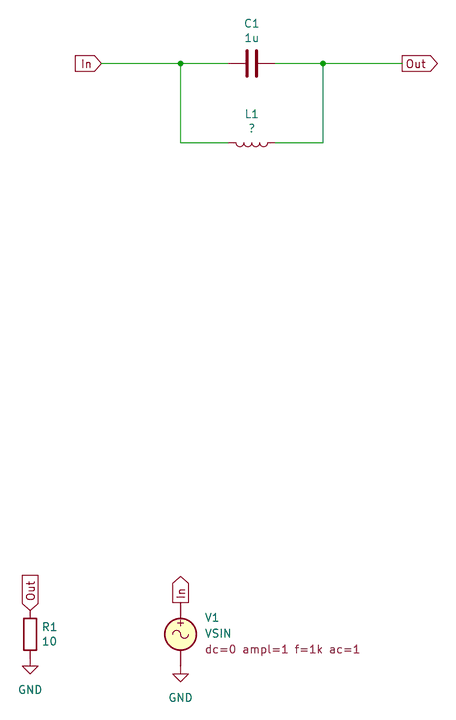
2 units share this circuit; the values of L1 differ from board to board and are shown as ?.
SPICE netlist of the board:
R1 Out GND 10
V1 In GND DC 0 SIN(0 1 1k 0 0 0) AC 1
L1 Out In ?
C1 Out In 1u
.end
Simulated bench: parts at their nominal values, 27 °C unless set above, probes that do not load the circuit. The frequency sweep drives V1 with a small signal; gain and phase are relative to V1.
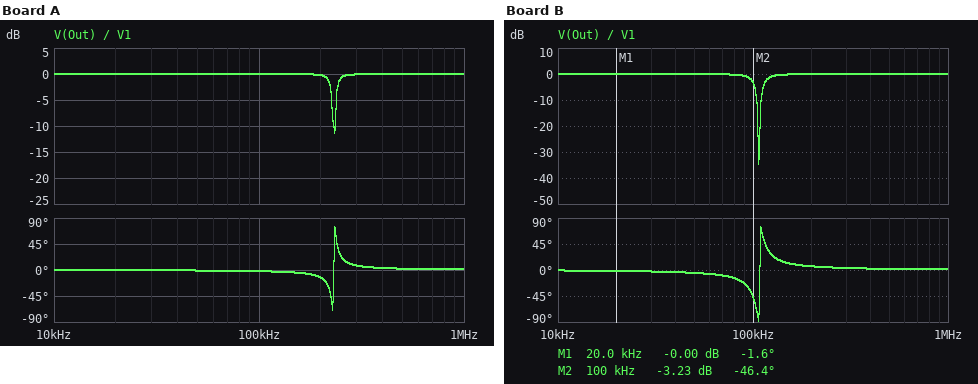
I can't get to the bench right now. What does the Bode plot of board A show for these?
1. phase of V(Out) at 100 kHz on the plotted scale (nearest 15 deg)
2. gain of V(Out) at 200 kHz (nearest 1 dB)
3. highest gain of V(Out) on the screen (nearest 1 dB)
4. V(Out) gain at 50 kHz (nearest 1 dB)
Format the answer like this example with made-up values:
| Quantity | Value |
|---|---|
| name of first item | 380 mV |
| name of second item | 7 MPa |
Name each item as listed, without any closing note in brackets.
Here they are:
| Quantity | Value |
|---|---|
| phase of V(Out) at 100 kHz on the plotted scale | 0 deg |
| gain of V(Out) at 200 kHz | 0 dB |
| highest gain of V(Out) on the screen | 0 dB |
| V(Out) gain at 50 kHz | 0 dB |
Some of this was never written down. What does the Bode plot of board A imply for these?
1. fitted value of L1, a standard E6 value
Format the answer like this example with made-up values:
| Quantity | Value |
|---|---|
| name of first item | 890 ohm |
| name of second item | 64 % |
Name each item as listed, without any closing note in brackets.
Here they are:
| Quantity | Value |
|---|---|
| fitted value of L1, a standard E6 value | 470 nH |
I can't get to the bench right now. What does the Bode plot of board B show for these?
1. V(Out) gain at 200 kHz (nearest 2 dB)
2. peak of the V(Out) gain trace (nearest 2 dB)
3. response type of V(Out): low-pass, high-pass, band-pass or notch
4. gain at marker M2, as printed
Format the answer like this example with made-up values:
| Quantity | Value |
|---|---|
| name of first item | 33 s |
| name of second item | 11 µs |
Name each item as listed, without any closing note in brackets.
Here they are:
| Quantity | Value |
|---|---|
| V(Out) gain at 200 kHz | 0 dB |
| peak of the V(Out) gain trace | 0 dB |
| response type of V(Out): low-pass, high-pass, band-pass or notch | notch |
| gain at marker M2, as printed | -3.23 dB |
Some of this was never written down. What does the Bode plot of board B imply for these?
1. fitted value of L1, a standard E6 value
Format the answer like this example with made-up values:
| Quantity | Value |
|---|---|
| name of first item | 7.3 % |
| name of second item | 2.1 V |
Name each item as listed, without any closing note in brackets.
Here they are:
| Quantity | Value |
|---|---|
| fitted value of L1, a standard E6 value | 2.2 µH |
